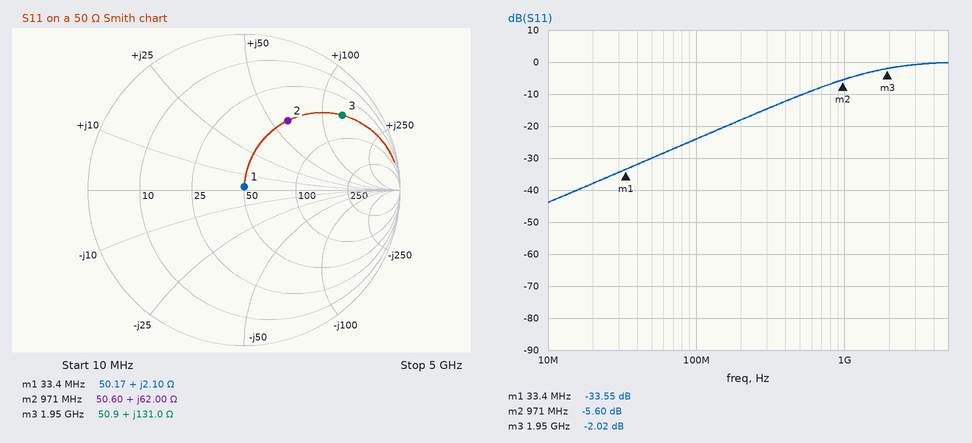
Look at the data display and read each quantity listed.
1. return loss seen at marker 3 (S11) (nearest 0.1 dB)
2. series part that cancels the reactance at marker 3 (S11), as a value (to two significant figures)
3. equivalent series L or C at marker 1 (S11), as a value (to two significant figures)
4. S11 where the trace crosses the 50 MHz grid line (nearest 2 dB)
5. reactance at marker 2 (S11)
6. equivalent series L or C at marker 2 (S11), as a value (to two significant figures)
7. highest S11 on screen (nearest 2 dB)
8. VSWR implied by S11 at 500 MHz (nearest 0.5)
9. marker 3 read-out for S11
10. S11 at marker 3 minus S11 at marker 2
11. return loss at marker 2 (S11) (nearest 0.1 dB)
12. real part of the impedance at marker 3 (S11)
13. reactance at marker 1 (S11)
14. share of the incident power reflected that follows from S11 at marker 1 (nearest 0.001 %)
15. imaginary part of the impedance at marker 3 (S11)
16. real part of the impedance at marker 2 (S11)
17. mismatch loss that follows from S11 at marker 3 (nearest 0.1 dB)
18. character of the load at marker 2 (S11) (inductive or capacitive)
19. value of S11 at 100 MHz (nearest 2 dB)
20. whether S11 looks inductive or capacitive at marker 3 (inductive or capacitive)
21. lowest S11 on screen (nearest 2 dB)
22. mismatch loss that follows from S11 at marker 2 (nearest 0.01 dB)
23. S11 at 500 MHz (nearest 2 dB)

2.0 dB
620 fF
10 nH
-30 dB
+62.00 Ω
10 nH
0 dB
2.0
-2.02 dB
3.58 dB
5.6 dB
50.9 Ω
+2.10 Ω
0.044 %
+131.0 Ω
50.60 Ω
4.3 dB
inductive
-24 dB
inductive
-44 dB
1.40 dB
-10 dB
